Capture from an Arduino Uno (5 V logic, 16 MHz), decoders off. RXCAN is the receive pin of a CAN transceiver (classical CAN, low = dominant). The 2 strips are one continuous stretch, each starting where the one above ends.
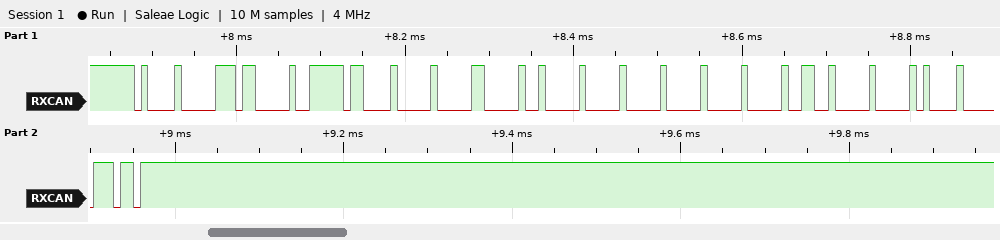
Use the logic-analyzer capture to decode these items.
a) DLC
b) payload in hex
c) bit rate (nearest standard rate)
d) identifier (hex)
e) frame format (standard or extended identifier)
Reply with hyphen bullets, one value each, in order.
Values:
- 8
- 01 01 00 00 00 00 C8 00
- 125 kbit/s
- 0x108180FE
- extended
